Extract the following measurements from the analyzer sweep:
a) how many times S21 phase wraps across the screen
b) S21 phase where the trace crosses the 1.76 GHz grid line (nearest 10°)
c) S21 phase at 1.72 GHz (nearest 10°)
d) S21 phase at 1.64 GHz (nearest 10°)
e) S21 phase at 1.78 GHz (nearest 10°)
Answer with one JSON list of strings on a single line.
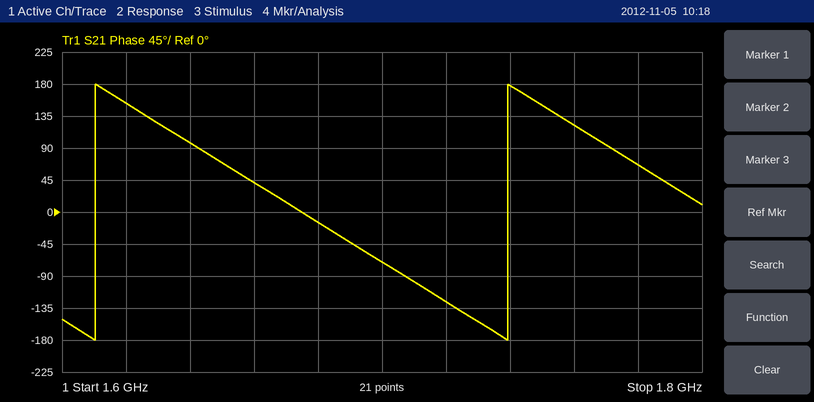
["2", "120°", "-130°", "100°", "70°"]
